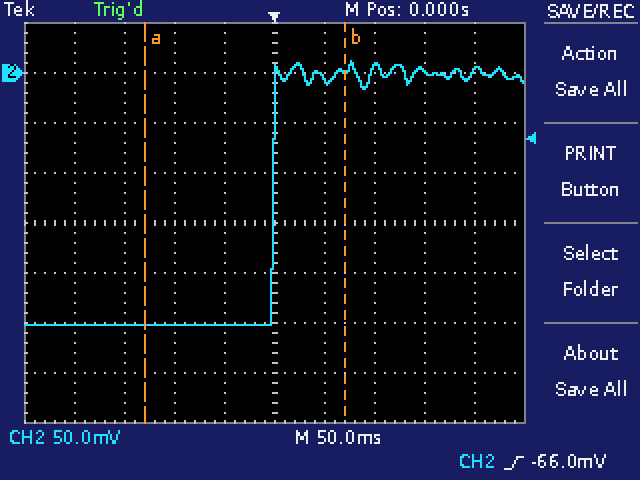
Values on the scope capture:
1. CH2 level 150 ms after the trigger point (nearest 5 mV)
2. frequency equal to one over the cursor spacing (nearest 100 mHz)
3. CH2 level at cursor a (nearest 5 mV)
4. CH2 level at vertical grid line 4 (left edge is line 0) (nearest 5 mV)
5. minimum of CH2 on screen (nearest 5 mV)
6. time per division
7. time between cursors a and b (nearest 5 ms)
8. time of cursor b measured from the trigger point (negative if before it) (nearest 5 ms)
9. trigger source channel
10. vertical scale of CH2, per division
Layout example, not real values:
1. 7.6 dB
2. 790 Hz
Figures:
1. 0 mV
2. 5.0 Hz
3. -250 mV
4. -250 mV
5. -250 mV
6. 50 ms
7. 200 ms
8. +70 ms
9. CH2
10. 50 mV
